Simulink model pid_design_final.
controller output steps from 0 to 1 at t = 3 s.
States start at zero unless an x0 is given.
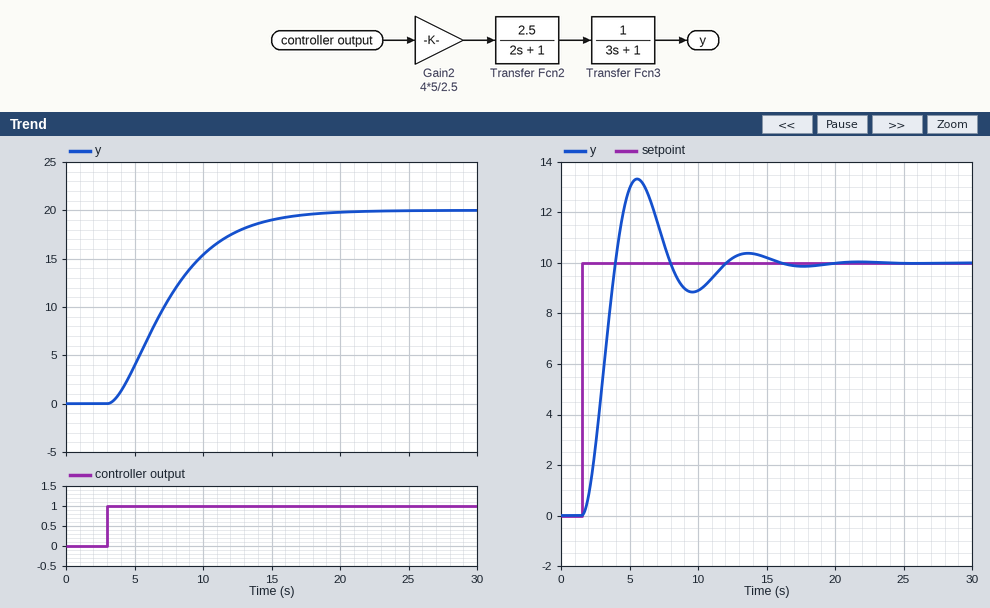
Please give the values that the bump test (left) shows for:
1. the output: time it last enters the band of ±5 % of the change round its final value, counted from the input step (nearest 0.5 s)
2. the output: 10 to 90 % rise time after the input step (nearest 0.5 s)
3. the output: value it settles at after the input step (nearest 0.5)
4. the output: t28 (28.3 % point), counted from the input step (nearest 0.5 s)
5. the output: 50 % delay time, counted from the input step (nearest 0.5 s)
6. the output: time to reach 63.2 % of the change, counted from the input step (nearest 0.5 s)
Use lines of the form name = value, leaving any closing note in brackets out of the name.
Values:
the output: time it last enters the band of ±5 % of the change round its final value, counted from the input step = 12.0 s
the output: 10 to 90 % rise time after the input step = 8.5 s
the output: value it settles at after the input step = 20.0
the output: t28 (28.3 % point), counted from the input step = 2.5 s
the output: 50 % delay time, counted from the input step = 4.0 s
the output: time to reach 63.2 % of the change, counted from the input step = 5.5 s
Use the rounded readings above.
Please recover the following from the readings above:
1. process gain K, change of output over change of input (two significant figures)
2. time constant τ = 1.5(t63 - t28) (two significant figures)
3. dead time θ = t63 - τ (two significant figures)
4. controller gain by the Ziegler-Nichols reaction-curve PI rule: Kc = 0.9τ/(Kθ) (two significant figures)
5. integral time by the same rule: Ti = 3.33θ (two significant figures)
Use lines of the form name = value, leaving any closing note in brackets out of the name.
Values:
process gain K, change of output over change of input = 20
time constant τ = 1.5(t63 - t28) = 4.5 s
dead time θ = t63 - τ = 1.0 s
controller gain by the Ziegler-Nichols reaction-curve PI rule: Kc = 0.9τ/(Kθ) = 0.20
integral time by the same rule: Ti = 3.33θ = 3.3 s
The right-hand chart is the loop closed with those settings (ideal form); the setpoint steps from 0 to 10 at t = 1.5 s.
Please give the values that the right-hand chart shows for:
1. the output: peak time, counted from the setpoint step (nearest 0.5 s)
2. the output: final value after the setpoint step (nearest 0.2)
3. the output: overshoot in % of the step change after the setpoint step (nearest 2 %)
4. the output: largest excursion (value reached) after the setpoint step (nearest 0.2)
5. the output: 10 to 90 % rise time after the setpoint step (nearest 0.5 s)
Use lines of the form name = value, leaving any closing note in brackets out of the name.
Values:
the output: peak time, counted from the setpoint step = 4.0 s
the output: final value after the setpoint step = 10.0
the output: overshoot in % of the step change after the setpoint step = 34 %
the output: largest excursion (value reached) after the setpoint step = 13.4
the output: 10 to 90 % rise time after the setpoint step = 1.5 s
